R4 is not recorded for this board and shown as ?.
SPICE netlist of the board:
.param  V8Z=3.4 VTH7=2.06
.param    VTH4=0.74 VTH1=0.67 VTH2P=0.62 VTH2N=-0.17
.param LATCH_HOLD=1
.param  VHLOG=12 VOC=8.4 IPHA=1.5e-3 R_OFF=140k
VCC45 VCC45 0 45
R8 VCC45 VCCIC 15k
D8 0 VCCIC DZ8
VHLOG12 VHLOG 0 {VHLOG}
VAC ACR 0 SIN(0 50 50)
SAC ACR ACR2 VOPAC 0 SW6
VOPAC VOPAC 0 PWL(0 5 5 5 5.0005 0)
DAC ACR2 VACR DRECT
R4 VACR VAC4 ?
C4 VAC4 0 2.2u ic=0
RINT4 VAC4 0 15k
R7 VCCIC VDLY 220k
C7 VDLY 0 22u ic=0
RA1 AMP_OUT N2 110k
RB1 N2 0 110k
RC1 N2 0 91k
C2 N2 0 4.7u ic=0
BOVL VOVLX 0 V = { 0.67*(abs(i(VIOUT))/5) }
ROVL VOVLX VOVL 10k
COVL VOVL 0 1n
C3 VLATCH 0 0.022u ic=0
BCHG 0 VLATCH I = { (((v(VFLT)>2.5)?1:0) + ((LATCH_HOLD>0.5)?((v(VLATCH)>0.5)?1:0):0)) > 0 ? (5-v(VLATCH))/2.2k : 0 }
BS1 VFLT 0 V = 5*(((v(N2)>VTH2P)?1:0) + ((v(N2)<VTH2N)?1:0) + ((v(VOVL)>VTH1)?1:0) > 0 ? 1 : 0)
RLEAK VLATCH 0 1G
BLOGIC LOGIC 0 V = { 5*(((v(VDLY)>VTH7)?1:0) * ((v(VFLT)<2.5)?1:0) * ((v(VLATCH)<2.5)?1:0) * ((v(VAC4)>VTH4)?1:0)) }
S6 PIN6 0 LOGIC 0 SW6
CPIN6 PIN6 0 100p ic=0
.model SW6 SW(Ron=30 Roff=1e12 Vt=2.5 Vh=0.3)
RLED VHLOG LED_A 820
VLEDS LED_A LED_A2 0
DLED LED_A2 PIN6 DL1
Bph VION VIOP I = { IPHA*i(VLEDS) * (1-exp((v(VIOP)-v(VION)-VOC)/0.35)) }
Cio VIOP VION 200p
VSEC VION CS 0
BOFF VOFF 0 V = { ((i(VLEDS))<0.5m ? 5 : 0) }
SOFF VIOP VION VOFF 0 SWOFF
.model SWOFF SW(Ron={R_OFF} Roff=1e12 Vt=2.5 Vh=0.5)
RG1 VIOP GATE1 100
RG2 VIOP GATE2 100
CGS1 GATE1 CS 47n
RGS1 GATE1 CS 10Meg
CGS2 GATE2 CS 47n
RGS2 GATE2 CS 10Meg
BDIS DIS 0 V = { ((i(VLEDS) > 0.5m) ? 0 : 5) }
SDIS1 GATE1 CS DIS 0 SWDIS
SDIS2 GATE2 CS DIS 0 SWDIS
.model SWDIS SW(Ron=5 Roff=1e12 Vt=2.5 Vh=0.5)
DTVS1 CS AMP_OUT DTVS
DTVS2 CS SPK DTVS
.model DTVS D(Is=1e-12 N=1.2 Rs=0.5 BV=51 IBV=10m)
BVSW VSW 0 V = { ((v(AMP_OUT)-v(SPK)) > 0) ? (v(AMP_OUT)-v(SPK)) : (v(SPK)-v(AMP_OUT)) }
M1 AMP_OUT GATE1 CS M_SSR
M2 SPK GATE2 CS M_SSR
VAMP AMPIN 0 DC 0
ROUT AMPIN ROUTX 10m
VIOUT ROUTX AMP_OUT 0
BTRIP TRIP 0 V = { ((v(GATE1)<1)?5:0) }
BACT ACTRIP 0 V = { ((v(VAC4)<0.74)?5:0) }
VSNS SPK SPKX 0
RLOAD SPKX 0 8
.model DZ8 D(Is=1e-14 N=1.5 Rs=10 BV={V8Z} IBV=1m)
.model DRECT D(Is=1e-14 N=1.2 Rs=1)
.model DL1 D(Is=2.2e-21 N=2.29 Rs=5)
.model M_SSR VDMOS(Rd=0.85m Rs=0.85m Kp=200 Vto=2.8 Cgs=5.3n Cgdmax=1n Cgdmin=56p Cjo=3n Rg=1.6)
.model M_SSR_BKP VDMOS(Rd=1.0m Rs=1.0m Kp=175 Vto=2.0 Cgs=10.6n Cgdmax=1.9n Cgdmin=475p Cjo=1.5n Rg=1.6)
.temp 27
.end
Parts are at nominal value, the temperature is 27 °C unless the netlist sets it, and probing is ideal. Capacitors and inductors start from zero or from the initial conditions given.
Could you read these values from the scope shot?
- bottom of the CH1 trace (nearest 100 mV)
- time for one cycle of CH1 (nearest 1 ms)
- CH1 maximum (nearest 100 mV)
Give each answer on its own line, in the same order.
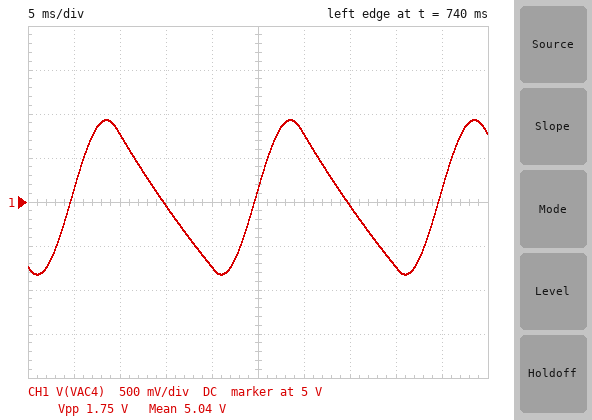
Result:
4.2 V
20 ms
5.9 V
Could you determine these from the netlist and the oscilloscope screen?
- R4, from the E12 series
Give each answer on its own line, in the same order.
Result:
39 kΩ
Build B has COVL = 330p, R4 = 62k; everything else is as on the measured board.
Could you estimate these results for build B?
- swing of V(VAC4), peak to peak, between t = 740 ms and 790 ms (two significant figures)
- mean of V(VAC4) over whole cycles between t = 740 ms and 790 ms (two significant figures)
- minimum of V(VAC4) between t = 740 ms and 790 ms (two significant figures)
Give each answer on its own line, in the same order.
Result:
1.2 V
3.4 V
2.8 V
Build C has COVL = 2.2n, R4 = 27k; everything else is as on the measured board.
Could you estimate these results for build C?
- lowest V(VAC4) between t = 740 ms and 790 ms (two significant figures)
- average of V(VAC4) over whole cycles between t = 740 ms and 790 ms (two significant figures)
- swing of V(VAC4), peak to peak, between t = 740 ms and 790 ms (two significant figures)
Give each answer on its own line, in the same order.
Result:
5.6 V
6.8 V
2.4 V
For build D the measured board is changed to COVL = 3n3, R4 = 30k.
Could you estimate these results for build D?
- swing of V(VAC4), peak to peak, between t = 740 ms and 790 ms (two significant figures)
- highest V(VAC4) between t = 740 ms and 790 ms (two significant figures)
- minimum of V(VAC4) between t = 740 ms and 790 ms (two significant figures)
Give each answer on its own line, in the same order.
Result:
2.2 V
7.4 V
5.2 V
